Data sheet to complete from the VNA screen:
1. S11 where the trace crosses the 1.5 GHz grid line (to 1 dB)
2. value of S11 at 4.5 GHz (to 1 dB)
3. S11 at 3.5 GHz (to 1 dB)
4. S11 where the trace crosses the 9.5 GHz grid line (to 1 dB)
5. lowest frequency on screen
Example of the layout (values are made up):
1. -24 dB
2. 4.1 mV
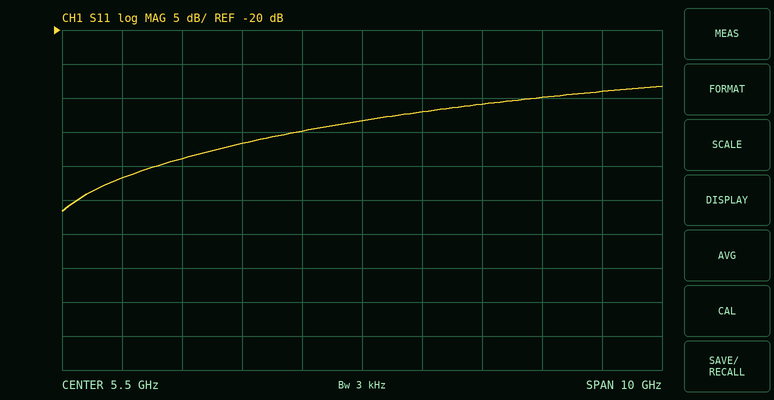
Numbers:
1. -42 dB
2. -35 dB
3. -37 dB
4. -29 dB
5. 500 MHz
